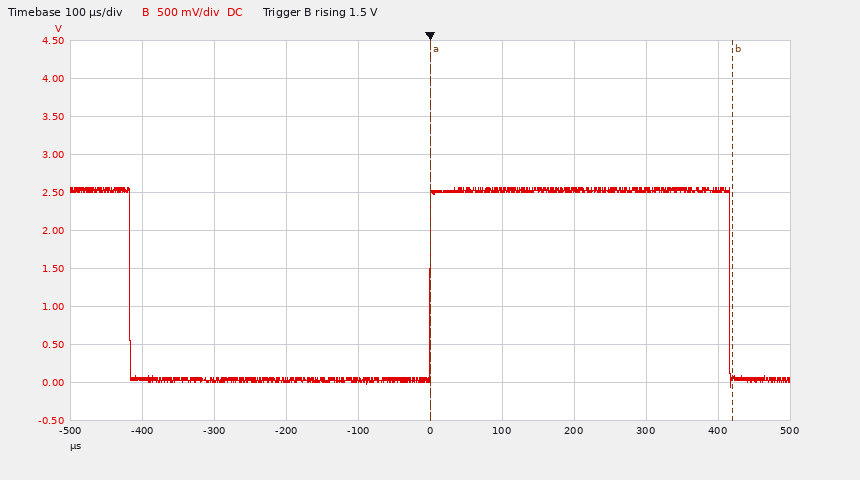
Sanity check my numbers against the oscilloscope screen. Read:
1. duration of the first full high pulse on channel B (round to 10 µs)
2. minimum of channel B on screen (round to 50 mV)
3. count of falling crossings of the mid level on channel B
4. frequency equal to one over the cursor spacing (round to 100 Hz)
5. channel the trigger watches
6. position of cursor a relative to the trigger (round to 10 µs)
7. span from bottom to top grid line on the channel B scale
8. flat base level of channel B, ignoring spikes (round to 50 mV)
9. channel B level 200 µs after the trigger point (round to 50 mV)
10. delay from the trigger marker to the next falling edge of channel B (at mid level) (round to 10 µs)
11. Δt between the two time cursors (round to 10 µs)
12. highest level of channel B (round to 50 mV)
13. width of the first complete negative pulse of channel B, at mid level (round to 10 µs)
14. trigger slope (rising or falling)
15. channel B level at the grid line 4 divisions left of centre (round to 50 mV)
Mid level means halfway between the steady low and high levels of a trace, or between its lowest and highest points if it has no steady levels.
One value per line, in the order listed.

420 µs
-50 mV
2
2.4 kHz
channel B
0 µs
5 V
50 mV
2.55 V
420 µs
420 µs
2.55 V
420 µs
rising
50 mV
